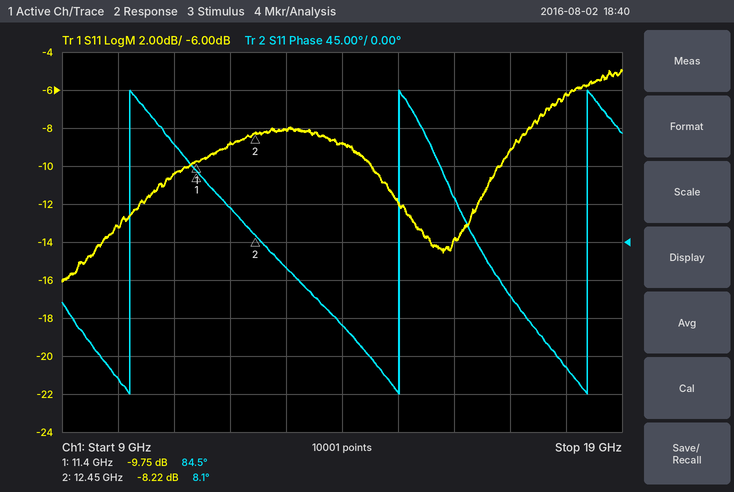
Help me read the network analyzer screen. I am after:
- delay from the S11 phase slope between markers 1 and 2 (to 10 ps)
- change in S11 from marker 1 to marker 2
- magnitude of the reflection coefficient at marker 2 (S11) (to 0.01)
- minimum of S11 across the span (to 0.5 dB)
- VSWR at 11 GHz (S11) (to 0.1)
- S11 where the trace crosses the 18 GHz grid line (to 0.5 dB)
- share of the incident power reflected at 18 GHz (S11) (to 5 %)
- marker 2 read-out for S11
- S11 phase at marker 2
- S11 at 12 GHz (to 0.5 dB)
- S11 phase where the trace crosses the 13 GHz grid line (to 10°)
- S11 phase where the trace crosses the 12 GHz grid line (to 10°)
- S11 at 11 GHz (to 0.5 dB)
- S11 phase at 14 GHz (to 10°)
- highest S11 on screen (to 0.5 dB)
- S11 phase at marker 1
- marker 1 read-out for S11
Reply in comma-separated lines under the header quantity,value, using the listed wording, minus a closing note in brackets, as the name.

quantity,value
delay from the S11 phase slope between markers 1 and 2,200 ps
change in S11 from marker 1 to marker 2,1.53 dB
magnitude of the reflection coefficient at marker 2 (S11),0.39
minimum of S11 across the span,-16.0 dB
VSWR at 11 GHz (S11),1.9
S11 where the trace crosses the 18 GHz grid line,-6.0 dB
share of the incident power reflected at 18 GHz (S11),25 %
marker 2 read-out for S11,-8.22 dB
S11 phase at marker 2,8.1°
S11 at 12 GHz,-9.0 dB
S11 phase where the trace crosses the 13 GHz grid line,-30°
S11 phase where the trace crosses the 12 GHz grid line,40°
S11 at 11 GHz,-10.5 dB
S11 phase at 14 GHz,-100°
highest S11 on screen,-5.0 dB
S11 phase at marker 1,84.5°
marker 1 read-out for S11,-9.75 dB
